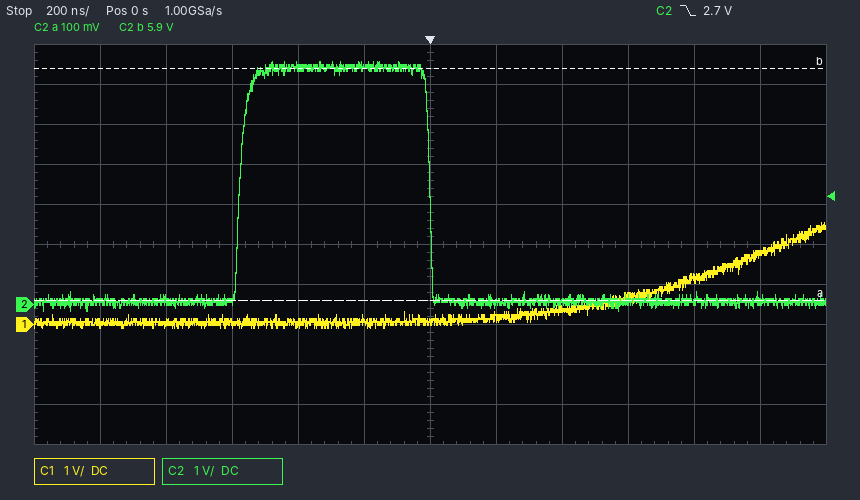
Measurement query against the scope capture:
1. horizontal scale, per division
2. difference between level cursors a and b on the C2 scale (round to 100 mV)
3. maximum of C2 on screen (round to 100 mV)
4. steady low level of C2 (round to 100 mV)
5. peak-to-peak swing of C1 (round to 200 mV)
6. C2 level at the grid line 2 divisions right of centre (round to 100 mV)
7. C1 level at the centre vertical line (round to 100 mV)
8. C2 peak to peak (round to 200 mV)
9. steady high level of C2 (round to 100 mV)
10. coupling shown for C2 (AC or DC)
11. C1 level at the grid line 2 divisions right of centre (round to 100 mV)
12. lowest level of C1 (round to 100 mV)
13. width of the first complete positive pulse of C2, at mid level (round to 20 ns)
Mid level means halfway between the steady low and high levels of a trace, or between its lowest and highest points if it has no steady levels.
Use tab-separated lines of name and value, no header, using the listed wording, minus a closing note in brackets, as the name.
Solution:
horizontal scale, per division	200 ns
difference between level cursors a and b on the C2 scale	5.8 V
maximum of C2 on screen	6.1 V
steady low level of C2	100 mV
peak-to-peak swing of C1	2.6 V
C2 level at the grid line 2 divisions right of centre	100 mV
C1 level at the centre vertical line	100 mV
C2 peak to peak	6.2 V
steady high level of C2	5.9 V
coupling shown for C2	DC
C1 level at the grid line 2 divisions right of centre	400 mV
lowest level of C1	-100 mV
width of the first complete positive pulse of C2, at mid level	580 ns
